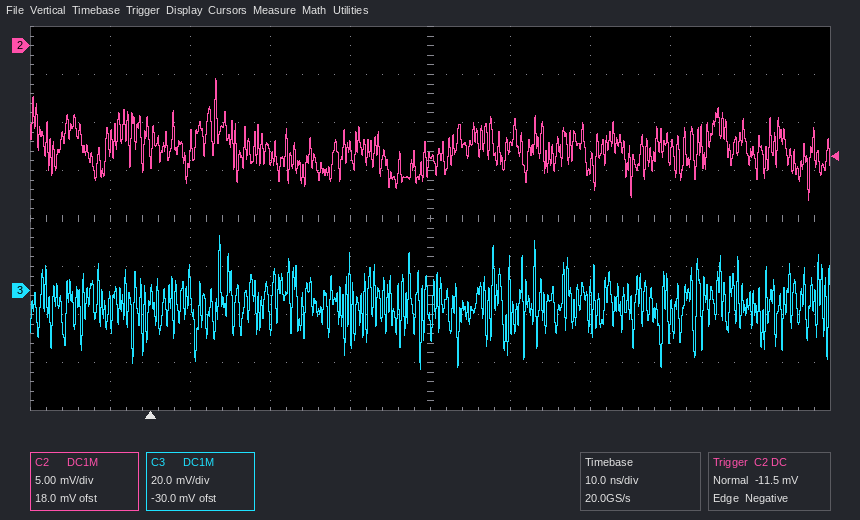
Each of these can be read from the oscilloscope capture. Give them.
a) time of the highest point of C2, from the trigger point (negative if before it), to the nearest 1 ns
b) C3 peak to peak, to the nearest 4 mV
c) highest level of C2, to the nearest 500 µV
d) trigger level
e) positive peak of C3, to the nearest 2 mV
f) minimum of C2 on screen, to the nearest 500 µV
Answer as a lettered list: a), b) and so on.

a) +8 ns
b) 56 mV
c) -3.5 mV
d) -11.5 mV
e) 22 mV
f) -16.0 mV
